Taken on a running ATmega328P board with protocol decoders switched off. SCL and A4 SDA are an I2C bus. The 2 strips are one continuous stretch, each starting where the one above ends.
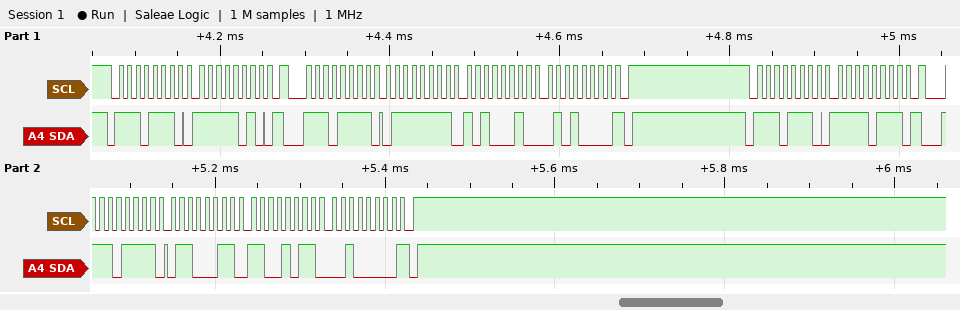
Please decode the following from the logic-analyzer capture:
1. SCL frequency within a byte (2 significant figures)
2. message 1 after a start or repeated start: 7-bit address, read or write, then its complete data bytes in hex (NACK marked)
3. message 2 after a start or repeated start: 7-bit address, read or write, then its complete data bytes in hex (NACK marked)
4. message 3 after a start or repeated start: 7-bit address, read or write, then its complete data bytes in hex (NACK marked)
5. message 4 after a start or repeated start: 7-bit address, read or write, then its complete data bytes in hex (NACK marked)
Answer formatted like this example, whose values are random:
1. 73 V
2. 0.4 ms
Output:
1. 100 kHz
2. 0x77 write: FA
3. 0x77 read: 7F A2 50 NACK
4. 0x77 write: F7
5. 0x77 read: 63 CB 20 NACK
